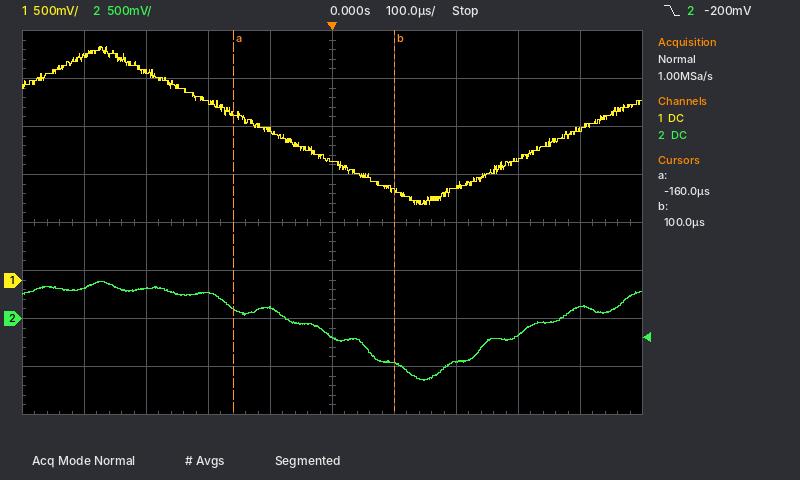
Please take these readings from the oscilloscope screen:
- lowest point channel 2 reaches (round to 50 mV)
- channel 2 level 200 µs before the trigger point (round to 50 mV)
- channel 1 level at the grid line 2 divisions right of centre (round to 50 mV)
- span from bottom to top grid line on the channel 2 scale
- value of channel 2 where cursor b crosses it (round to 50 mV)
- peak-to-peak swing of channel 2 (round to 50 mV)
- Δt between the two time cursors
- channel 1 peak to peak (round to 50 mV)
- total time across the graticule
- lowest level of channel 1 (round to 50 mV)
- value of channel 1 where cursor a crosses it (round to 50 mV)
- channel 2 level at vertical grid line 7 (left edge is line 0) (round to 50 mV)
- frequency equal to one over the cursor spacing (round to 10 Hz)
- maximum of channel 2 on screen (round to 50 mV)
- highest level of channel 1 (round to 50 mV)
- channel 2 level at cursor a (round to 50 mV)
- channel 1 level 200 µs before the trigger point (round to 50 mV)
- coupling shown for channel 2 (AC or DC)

-650 mV
250 mV
950 mV
4 V
-450 mV
1.05 V
260 µs
1.65 V
1 ms
800 mV
1.75 V
-450 mV
3.85 kHz
400 mV
2.45 V
100 mV
1.85 V
DC
